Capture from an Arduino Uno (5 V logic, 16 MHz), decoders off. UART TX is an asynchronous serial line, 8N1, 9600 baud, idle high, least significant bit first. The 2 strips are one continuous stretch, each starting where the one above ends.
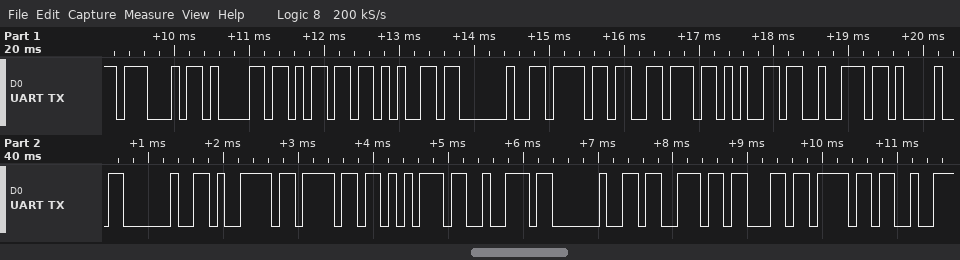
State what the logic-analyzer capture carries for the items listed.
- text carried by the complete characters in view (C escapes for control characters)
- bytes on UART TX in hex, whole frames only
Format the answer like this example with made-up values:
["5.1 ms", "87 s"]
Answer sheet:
["\"Game over! your sco\"", "47 61 6D 65 20 6F 76 65 72 21 20 79 6F 75 72 20 73 63 6F"]
